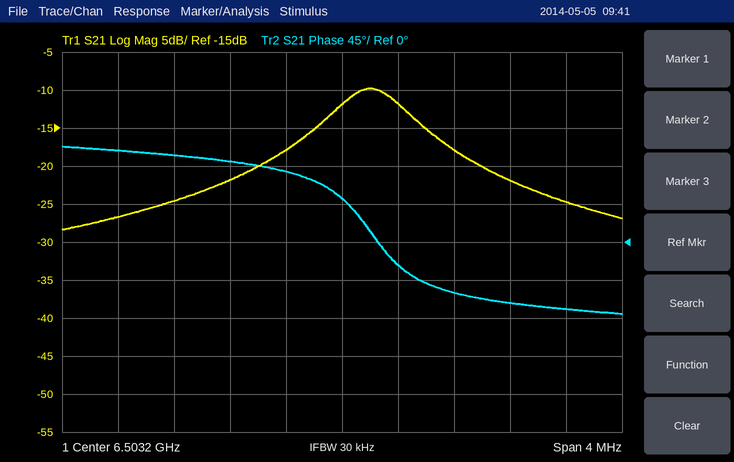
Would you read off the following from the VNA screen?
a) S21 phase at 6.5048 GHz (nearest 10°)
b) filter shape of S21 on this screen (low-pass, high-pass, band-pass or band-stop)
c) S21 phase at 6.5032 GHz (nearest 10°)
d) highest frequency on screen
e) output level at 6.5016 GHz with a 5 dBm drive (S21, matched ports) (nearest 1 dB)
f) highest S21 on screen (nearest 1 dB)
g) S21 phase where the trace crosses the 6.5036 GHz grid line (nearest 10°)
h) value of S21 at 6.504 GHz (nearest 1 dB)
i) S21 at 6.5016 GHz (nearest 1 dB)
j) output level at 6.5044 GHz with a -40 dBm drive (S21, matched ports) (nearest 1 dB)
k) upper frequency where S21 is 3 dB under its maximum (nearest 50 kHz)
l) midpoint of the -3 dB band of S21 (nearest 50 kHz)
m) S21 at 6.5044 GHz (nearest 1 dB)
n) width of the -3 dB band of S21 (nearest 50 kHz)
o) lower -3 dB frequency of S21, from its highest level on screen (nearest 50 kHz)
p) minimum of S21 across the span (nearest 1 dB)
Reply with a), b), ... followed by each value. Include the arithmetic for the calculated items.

a) -80°
b) band-pass
c) 50°
d) 6.5052 GHz
e) 5 dBm + (-27 dB) = -22 dBm
f) -10 dB
g) -30°
h) -18 dB
i) -27 dB
j) -40 dBm + (-22 dB) = -62 dBm
k) 6.50365 GHz
l) 6.50340 GHz
m) -22 dB
n) 6.50365 GHz − 6.50315 GHz = 500 kHz
o) 6.50315 GHz
p) -28 dB
